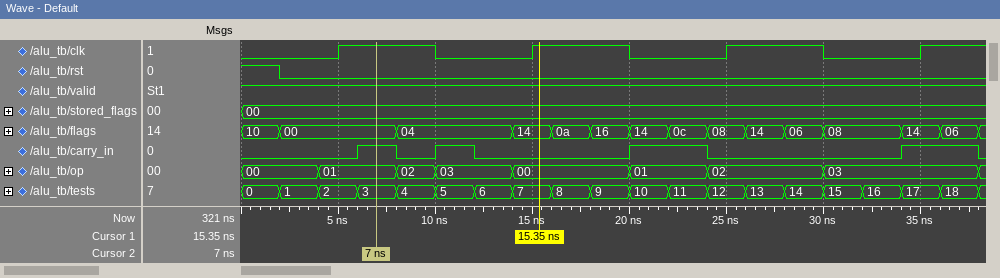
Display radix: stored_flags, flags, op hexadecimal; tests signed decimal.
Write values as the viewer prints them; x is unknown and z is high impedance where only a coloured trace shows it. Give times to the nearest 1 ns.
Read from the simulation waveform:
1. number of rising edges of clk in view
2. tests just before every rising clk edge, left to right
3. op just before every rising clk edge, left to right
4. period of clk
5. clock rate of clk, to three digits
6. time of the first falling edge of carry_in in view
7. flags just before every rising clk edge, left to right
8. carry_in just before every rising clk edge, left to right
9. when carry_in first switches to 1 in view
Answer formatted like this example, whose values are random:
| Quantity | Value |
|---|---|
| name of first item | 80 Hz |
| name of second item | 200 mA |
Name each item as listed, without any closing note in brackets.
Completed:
| Quantity | Value |
|---|---|
| number of rising edges of clk in view | 4 |
| tests just before every rising clk edge, left to right | 2, 7, 12, 17 |
| op just before every rising clk edge, left to right | 01, 00, 02, 03 |
| period of clk | 10 ns |
| clock rate of clk, to three digits | 100 MHz |
| time of the first falling edge of carry_in in view | 8 ns |
| flags just before every rising clk edge, left to right | 00, 14, 08, 14 |
| carry_in just before every rising clk edge, left to right | 0 0 0 1 |
| when carry_in first switches to 1 in view | 6 ns |
